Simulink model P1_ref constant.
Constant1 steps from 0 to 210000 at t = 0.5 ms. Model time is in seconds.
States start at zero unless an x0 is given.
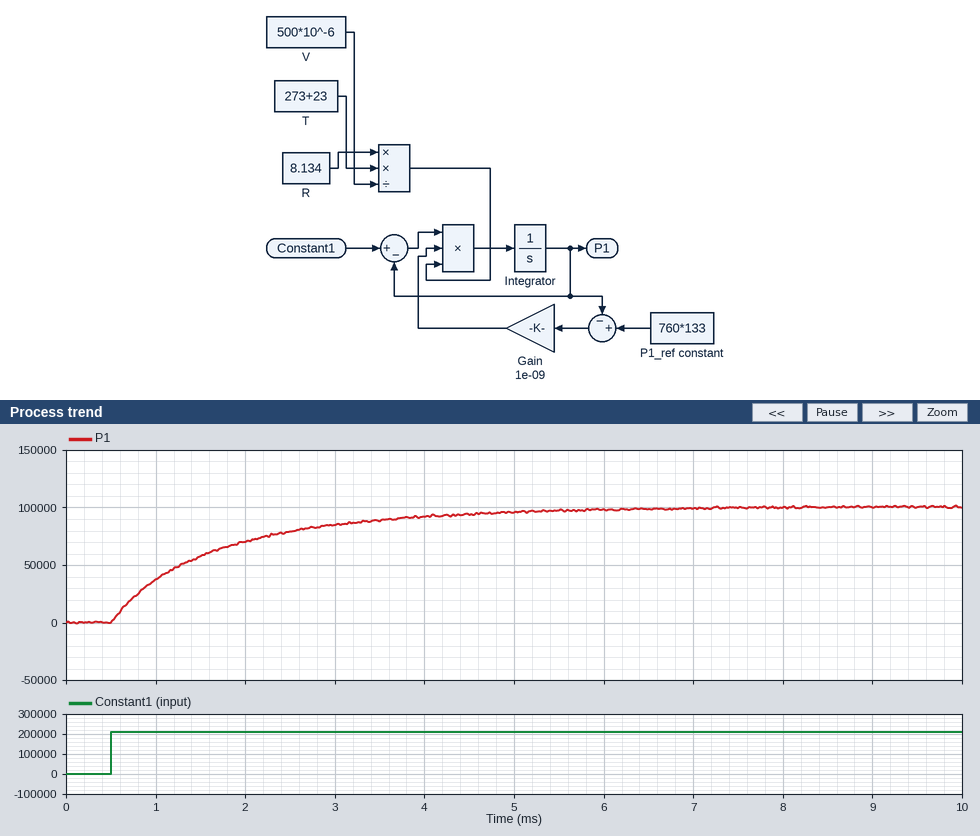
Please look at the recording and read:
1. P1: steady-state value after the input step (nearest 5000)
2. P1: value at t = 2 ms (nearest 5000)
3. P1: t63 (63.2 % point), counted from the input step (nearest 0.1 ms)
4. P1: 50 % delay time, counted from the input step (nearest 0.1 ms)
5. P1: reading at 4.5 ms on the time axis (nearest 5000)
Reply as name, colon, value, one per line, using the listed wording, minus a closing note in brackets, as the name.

P1: steady-state value after the input step: 100000
P1: value at t = 2 ms: 70000
P1: t63 (63.2 % point), counted from the input step: 1.2 ms
P1: 50 % delay time, counted from the input step: 0.8 ms
P1: reading at 4.5 ms on the time axis: 95000
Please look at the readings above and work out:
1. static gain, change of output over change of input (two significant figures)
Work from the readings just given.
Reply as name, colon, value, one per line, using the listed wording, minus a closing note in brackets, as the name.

static gain, change of output over change of input: 0.48
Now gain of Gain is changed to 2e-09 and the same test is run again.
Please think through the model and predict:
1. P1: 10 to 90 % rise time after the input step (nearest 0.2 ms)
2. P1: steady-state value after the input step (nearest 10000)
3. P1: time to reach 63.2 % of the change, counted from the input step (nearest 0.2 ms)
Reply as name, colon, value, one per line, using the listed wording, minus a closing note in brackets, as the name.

P1: 10 to 90 % rise time after the input step: 1.6 ms
P1: steady-state value after the input step: 100000
P1: time to reach 63.2 % of the change, counted from the input step: 0.6 ms
